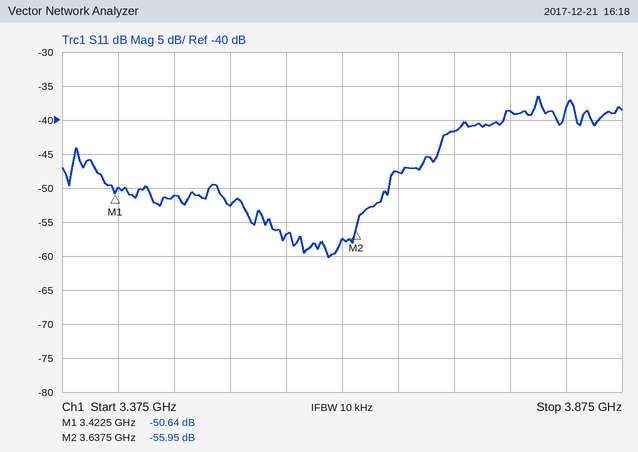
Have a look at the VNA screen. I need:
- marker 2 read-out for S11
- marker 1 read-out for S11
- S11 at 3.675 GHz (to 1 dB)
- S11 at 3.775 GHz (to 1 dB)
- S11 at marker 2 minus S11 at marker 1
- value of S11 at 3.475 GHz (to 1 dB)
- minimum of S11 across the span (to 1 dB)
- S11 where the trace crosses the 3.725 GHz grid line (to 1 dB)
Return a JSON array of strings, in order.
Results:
["-55.95 dB", "-50.64 dB", "-48 dB", "-39 dB", "-5.31 dB", "-51 dB", "-60 dB", "-42 dB"]
